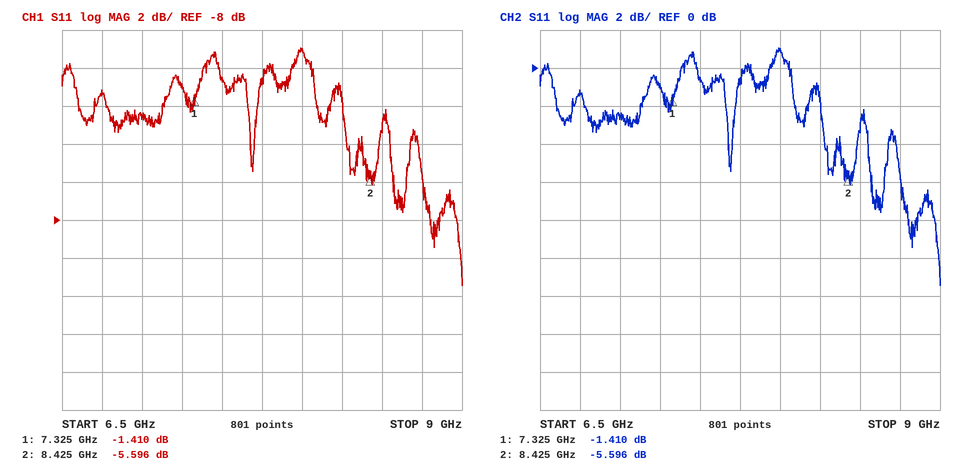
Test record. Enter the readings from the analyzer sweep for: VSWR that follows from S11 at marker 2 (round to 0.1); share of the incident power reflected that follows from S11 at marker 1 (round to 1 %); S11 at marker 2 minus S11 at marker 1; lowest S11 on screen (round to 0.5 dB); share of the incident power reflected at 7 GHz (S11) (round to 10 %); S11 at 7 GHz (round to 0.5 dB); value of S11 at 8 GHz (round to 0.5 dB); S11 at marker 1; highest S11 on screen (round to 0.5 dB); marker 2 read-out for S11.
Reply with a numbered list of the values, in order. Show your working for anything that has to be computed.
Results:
1. (1 + 0.5250)/(1 − 0.5250) ≈ 3.2
2. 10^(-1.41/10) ≈ 72 %
3. -5.596 − (-1.41) = -4.186 dB
4. -11.5 dB
5. 10^(-2.5/10) ≈ 56.2 %, so 60 % to the nearest 10 %
6. -2.5 dB
7. 1.0 dB
8. -1.410 dB
9. 1.0 dB
10. -5.596 dB
